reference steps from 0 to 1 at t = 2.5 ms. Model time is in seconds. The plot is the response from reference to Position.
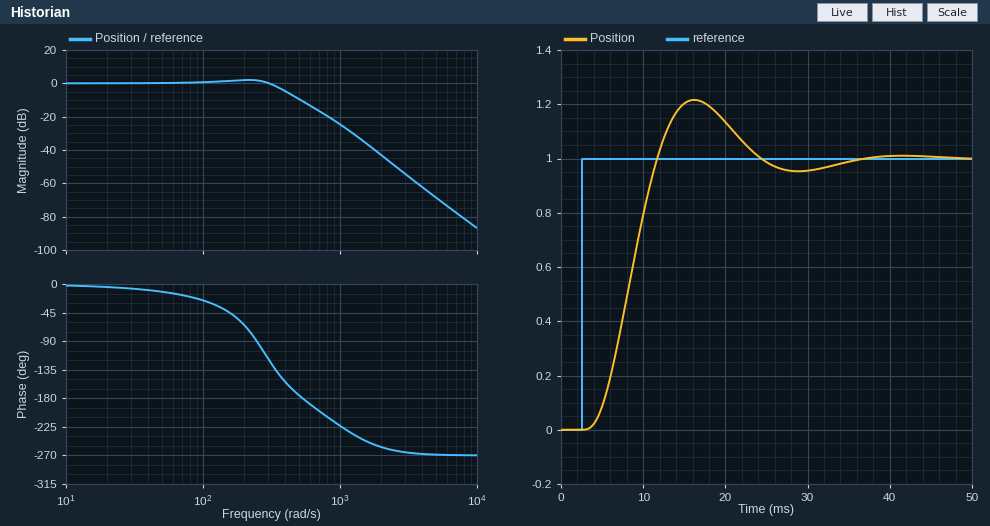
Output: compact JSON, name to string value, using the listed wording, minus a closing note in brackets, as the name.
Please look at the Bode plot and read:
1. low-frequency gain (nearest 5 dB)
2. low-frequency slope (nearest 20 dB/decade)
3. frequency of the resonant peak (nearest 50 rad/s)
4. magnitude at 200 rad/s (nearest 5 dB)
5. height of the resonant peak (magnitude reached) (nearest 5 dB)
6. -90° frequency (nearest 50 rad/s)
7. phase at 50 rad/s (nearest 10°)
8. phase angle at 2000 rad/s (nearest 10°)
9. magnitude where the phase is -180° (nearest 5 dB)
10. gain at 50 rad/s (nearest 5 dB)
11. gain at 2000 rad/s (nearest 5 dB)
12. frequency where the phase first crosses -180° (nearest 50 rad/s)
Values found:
{"low-frequency gain": "0 dB", "low-frequency slope": "0 dB/decade", "frequency of the resonant peak": "200 rad/s", "magnitude at 200 rad/s": "0 dB", "height of the resonant peak (magnitude reached)": "0 dB", "-90° frequency": "250 rad/s", "phase at 50 rad/s": "-10°", "phase angle at 2000 rad/s": "-260°", "magnitude where the phase is -180°": "-10 dB", "gain at 50 rad/s": "0 dB", "gain at 2000 rad/s": "-45 dB", "frequency where the phase first crosses -180°": "550 rad/s"}
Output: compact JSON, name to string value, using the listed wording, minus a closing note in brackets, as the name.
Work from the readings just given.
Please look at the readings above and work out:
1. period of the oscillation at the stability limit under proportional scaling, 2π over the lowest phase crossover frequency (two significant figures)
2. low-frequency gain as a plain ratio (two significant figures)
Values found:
{"period of the oscillation at the stability limit under proportional scaling, 2π over the lowest phase crossover frequency": "0.011 s", "low-frequency gain as a plain ratio": "1.0"}
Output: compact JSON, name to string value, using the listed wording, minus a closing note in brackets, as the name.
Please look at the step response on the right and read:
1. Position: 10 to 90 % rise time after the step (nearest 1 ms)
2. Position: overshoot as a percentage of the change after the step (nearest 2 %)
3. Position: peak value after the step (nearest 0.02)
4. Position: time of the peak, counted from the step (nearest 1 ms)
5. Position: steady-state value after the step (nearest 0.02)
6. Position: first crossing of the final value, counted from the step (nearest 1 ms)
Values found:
{"Position: 10 to 90 % rise time after the step": "6 ms", "Position: overshoot as a percentage of the change after the step": "22 %", "Position: peak value after the step": "1.22", "Position: time of the peak, counted from the step": "14 ms", "Position: steady-state value after the step": "1.00", "Position: first crossing of the final value, counted from the step": "9 ms"}
